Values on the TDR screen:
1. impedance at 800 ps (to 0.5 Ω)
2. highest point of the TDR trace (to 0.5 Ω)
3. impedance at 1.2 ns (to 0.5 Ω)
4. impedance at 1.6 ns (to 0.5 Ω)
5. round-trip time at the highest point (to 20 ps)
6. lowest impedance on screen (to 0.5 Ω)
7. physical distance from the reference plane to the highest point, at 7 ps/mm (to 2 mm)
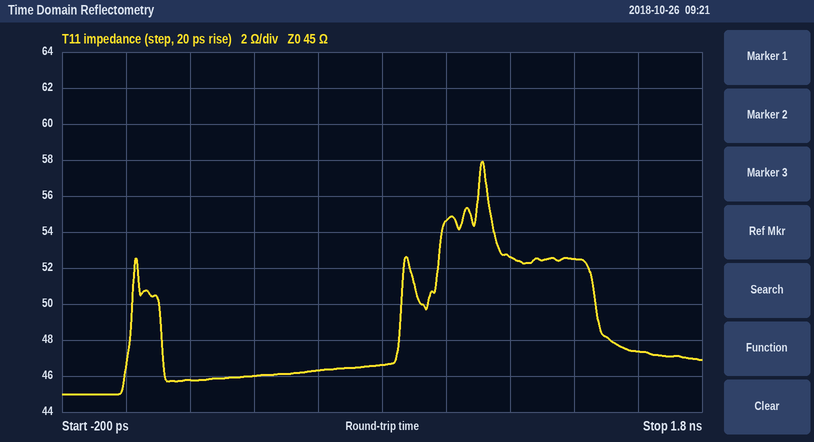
46.5 Ω
58.0 Ω
52.5 Ω
47.5 Ω
1.12 ns
45.0 Ω
80 mm
